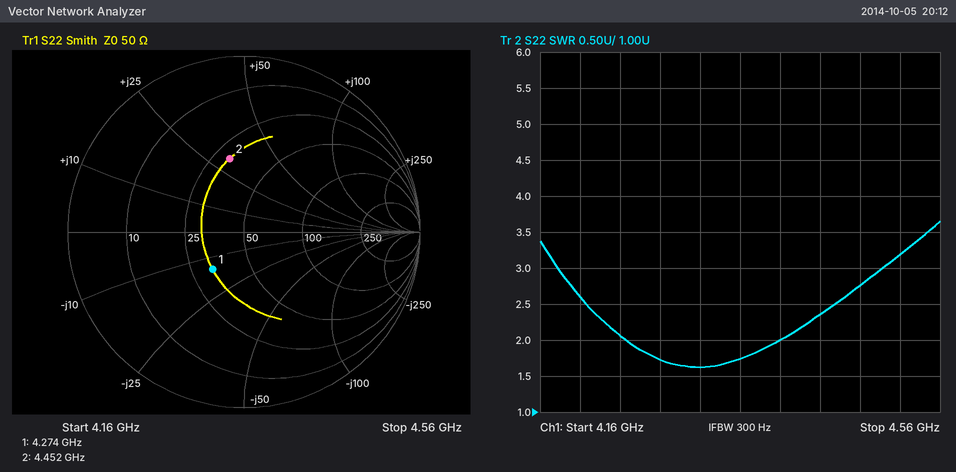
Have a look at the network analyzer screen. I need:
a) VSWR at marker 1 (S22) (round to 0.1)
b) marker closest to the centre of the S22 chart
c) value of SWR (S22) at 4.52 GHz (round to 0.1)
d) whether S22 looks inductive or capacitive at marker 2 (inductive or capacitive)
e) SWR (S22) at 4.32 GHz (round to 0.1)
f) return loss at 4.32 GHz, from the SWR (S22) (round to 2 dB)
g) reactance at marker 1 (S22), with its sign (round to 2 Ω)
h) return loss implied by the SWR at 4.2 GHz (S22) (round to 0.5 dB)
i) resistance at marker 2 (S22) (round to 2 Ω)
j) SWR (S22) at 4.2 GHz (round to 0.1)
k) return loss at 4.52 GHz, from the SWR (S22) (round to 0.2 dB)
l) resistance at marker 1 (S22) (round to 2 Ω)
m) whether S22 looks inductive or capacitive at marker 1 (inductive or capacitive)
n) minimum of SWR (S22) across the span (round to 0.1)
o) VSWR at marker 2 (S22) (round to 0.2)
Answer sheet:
1.8
marker 1
3.2
inductive
1.6
12 dB
-14 Ω
7.0 dB
30 Ω
2.6
5.6 dB
32 Ω
capacitive
1.6
2.4
